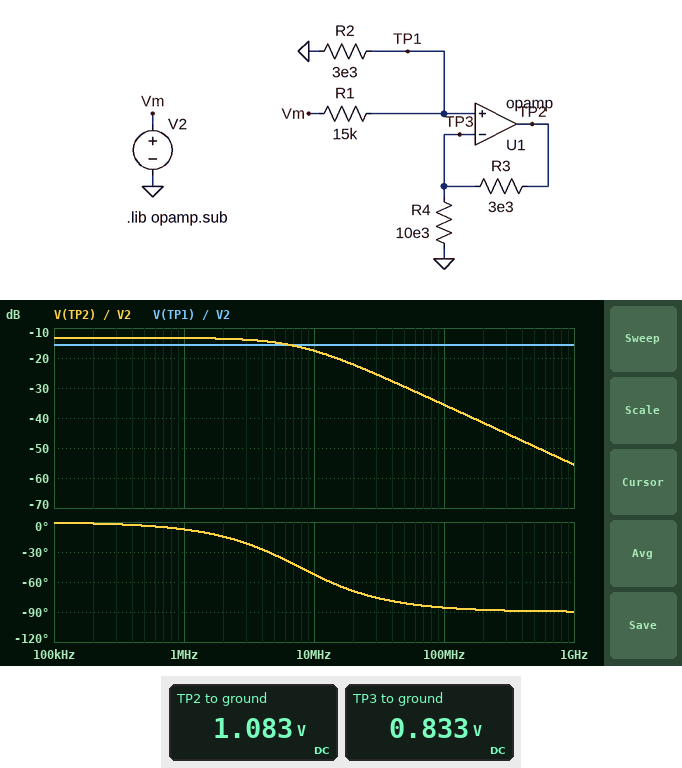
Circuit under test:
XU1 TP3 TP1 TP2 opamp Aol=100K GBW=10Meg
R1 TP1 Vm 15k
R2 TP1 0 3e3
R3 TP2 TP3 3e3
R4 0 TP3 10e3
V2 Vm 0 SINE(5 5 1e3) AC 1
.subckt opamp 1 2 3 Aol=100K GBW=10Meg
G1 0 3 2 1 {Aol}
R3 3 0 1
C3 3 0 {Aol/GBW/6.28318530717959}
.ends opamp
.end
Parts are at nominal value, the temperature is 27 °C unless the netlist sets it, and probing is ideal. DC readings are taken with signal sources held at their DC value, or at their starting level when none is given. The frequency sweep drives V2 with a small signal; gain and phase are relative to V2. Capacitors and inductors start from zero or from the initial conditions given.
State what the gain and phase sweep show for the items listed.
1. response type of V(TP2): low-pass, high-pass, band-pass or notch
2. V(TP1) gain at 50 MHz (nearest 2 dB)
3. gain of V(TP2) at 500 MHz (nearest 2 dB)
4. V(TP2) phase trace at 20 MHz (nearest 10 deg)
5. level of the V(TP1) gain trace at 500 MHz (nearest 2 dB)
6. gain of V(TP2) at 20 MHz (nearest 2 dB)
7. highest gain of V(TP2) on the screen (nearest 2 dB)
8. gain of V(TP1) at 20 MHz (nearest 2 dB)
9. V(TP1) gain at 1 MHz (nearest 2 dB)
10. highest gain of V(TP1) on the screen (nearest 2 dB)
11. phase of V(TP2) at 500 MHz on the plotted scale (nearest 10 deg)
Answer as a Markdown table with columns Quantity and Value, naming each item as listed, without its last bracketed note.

| Quantity | Value |
|---|---|
| response type of V(TP2): low-pass, high-pass, band-pass or notch | low-pass |
| V(TP1) gain at 50 MHz | -16 dB |
| gain of V(TP2) at 500 MHz | -50 dB |
| V(TP2) phase trace at 20 MHz | -70 deg |
| level of the V(TP1) gain trace at 500 MHz | -16 dB |
| gain of V(TP2) at 20 MHz | -22 dB |
| highest gain of V(TP2) on the screen | -14 dB |
| gain of V(TP1) at 20 MHz | -16 dB |
| V(TP1) gain at 1 MHz | -16 dB |
| highest gain of V(TP1) on the screen | -16 dB |
| phase of V(TP2) at 500 MHz on the plotted scale | -90 deg |
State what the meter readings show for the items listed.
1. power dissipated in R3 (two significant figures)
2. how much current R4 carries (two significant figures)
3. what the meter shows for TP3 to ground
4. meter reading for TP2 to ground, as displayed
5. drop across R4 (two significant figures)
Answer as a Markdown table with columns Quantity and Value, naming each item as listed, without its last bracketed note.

| Quantity | Value |
|---|---|
| power dissipated in R3 | 21 µW |
| how much current R4 carries | 83 µA |
| what the meter shows for TP3 to ground | 0.833 V |
| meter reading for TP2 to ground, as displayed | 1.083 V |
| drop across R4 | 830 mV |
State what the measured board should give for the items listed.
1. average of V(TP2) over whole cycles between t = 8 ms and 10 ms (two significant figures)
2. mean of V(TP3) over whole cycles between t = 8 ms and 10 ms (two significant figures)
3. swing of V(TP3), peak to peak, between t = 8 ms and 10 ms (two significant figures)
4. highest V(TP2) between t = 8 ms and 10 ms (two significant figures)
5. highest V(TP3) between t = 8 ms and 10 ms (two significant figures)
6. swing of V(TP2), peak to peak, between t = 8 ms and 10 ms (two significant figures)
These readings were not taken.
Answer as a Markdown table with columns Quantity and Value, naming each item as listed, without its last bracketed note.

| Quantity | Value |
|---|---|
| average of V(TP2) over whole cycles between t = 8 ms and 10 ms | 1.1 V |
| mean of V(TP3) over whole cycles between t = 8 ms and 10 ms | 830 mV |
| swing of V(TP3), peak to peak, between t = 8 ms and 10 ms | 1.7 V |
| highest V(TP2) between t = 8 ms and 10 ms | 2.2 V |
| highest V(TP3) between t = 8 ms and 10 ms | 1.7 V |
| swing of V(TP2), peak to peak, between t = 8 ms and 10 ms | 2.2 V |
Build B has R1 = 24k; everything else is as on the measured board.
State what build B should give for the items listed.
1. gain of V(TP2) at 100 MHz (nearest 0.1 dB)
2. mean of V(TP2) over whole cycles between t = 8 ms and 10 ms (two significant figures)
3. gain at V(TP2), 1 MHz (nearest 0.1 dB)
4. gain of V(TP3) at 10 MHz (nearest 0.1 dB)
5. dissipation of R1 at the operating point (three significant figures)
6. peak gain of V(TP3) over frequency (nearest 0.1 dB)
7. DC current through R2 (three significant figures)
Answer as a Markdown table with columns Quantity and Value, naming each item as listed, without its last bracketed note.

| Quantity | Value |
|---|---|
| gain of V(TP2) at 100 MHz | -39.1 dB |
| mean of V(TP2) over whole cycles between t = 8 ms and 10 ms | 720 mV |
| gain at V(TP2), 1 MHz | -16.9 dB |
| gain of V(TP3) at 10 MHz | -23.4 dB |
| dissipation of R1 at the operating point | 823 µW |
| peak gain of V(TP3) over frequency | -19.1 dB |
| DC current through R2 | 185 µA |
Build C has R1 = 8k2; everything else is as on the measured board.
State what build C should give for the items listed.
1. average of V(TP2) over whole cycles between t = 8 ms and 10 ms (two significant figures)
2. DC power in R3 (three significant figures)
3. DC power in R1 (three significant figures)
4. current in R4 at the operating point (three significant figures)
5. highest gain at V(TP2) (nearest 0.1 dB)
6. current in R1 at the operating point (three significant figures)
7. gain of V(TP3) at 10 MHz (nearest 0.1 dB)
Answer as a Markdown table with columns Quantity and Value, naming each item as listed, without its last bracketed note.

| Quantity | Value |
|---|---|
| average of V(TP2) over whole cycles between t = 8 ms and 10 ms | 1.7 V |
| DC power in R3 | 53.8 µW |
| DC power in R1 | 1.63 mW |
| current in R4 at the operating point | 134 µA |
| highest gain at V(TP2) | -9.2 dB |
| current in R1 at the operating point | 446 µA |
| gain of V(TP3) at 10 MHz | -15.7 dB |
